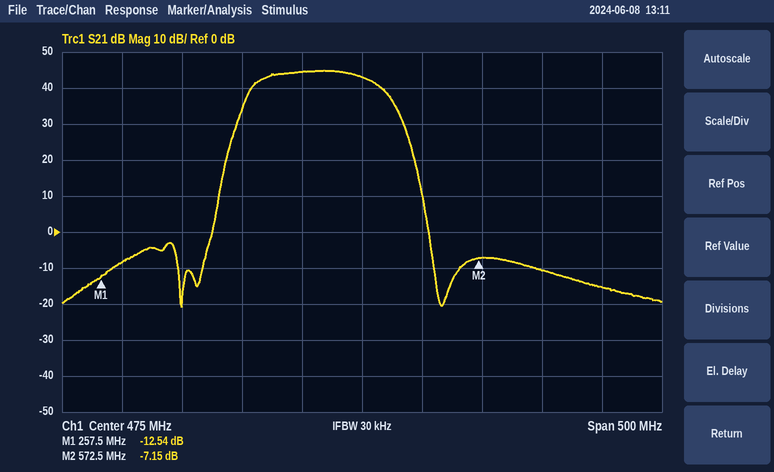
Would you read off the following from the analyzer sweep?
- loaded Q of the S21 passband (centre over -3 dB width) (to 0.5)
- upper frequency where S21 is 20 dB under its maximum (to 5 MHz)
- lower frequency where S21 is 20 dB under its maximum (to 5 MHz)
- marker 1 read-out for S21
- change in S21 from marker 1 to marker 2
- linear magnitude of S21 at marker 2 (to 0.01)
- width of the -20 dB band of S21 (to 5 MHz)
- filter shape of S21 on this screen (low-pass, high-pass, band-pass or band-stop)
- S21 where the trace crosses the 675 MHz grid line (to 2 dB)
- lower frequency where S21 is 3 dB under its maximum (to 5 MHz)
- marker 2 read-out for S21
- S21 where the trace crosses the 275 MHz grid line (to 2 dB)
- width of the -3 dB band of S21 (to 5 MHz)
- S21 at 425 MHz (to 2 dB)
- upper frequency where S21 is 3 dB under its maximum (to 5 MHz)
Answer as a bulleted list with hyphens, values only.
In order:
- 4.5
- 515 MHz
- 365 MHz
- -12.54 dB
- 5.39 dB
- 0.44
- 150 MHz
- band-pass
- -16 dB
- 390 MHz
- -7.15 dB
- -8 dB
- 95 MHz
- 44 dB
- 485 MHz
